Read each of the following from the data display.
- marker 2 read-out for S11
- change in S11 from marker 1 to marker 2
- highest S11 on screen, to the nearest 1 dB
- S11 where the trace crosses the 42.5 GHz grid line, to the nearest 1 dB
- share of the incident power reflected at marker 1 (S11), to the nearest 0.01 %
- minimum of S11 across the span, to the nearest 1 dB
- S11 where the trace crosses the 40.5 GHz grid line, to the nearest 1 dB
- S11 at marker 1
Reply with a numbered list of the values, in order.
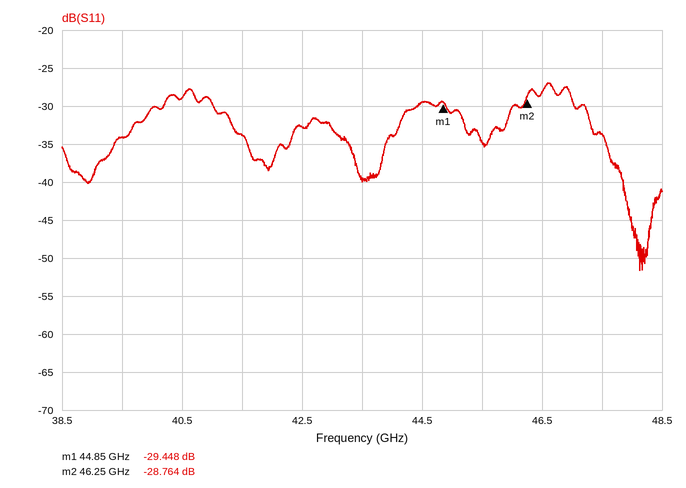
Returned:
1. -28.764 dB
2. 0.684 dB
3. -27 dB
4. -33 dB
5. 0.11 %
6. -52 dB
7. -29 dB
8. -29.448 dB
